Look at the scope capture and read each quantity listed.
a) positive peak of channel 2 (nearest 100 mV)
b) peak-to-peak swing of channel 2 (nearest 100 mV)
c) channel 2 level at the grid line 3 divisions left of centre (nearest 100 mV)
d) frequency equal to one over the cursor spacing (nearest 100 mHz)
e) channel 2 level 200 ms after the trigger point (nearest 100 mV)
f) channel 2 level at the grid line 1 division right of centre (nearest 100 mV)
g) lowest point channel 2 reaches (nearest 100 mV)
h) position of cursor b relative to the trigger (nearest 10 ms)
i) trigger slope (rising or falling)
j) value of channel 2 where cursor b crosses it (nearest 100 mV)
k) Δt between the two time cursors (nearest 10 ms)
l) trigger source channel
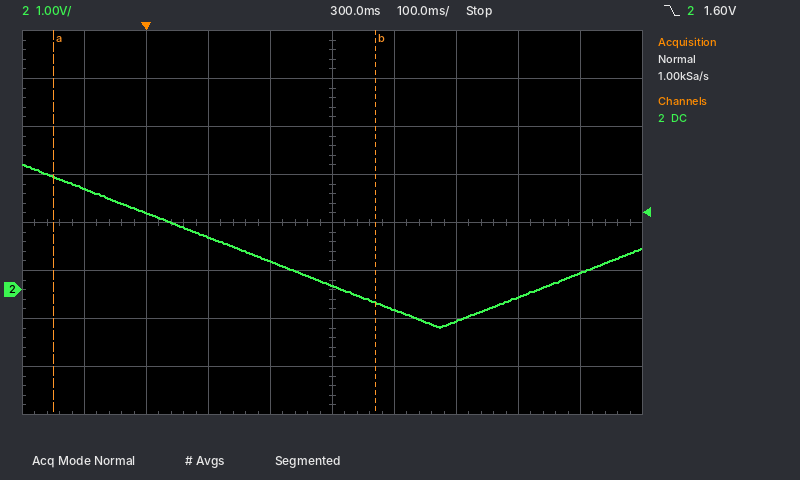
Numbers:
2.6 V
3.4 V
1.6 V
1.9 Hz
600 mV
-400 mV
-800 mV
+370 ms
falling
-300 mV
520 ms
channel 2
